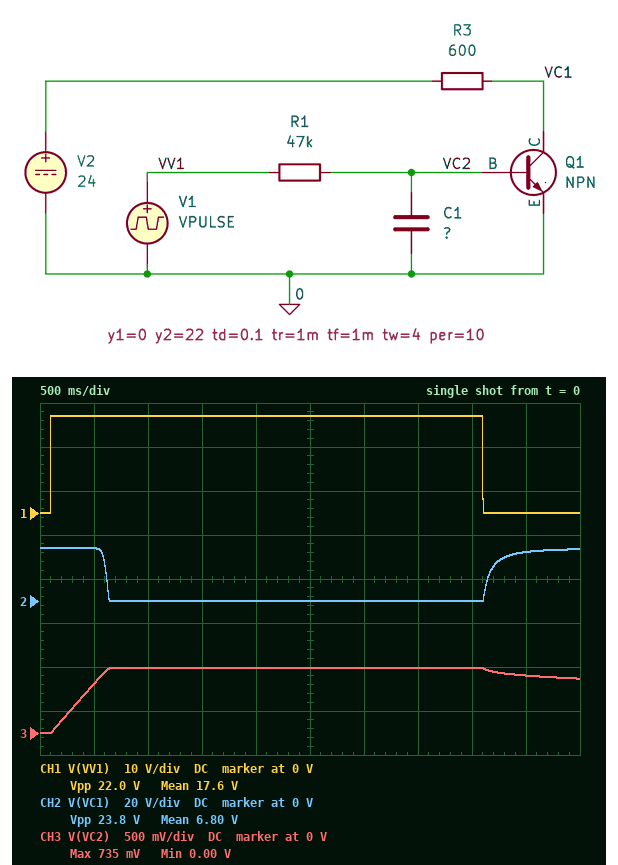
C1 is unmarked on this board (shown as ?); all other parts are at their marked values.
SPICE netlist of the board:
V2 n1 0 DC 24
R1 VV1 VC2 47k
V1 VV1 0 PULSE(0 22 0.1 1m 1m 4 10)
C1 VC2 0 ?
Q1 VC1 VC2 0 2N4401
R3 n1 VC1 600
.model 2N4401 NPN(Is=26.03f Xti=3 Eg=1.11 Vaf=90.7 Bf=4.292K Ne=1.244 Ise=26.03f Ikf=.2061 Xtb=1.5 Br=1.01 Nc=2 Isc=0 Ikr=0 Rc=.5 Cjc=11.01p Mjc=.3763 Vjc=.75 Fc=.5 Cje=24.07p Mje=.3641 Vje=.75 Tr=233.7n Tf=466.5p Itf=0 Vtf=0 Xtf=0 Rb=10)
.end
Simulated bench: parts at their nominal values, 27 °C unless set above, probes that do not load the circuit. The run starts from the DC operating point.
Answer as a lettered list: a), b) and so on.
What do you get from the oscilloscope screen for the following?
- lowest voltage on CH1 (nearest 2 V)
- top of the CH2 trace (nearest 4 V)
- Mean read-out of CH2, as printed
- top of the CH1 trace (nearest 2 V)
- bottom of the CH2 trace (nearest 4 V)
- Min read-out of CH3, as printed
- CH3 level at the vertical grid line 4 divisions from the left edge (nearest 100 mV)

a) 0 V
b) 24 V
c) 6.80 V
d) 22 V
e) 0 V
f) 0.00 V
g) 700 mV
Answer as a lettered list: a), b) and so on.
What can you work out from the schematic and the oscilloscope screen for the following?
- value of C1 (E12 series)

a) 330 µF
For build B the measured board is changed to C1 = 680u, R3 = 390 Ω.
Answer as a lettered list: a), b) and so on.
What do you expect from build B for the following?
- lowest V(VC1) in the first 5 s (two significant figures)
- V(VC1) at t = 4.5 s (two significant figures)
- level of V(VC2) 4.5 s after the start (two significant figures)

a) 190 mV
b) 21 V
c) 680 mV
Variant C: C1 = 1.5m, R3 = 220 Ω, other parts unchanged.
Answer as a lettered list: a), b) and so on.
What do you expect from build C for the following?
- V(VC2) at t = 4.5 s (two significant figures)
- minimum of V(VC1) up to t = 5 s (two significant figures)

a) 710 mV
b) 3.5 V
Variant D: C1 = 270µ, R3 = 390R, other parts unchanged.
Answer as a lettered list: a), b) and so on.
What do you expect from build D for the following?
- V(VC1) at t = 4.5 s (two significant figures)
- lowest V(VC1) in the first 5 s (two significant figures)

a) 23 V
b) 190 mV
